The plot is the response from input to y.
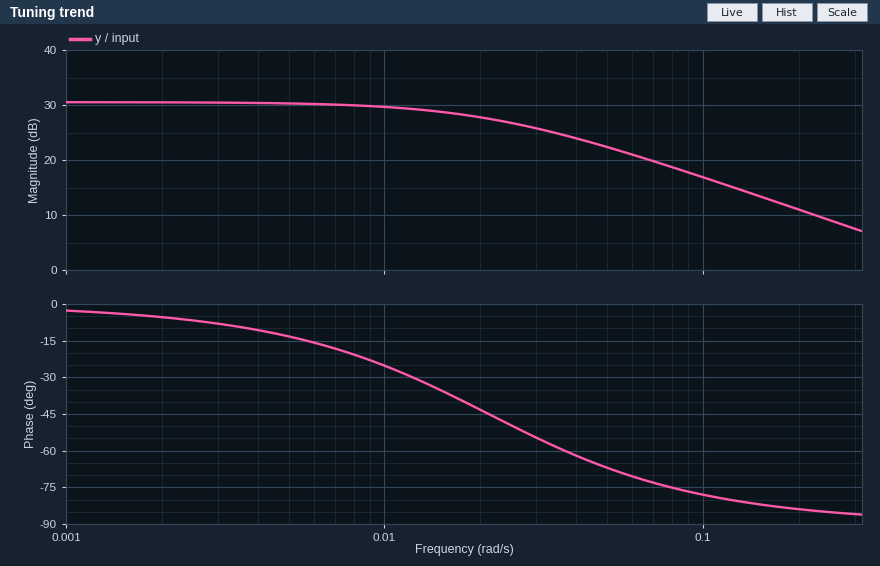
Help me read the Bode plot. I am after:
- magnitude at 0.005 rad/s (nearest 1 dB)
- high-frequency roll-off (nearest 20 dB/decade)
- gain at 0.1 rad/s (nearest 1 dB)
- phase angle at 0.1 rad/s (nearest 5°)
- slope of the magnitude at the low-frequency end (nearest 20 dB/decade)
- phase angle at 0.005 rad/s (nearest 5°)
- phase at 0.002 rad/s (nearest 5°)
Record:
30 dB
-20 dB/decade
17 dB
-80°
0 dB/decade
-15°
-5°
